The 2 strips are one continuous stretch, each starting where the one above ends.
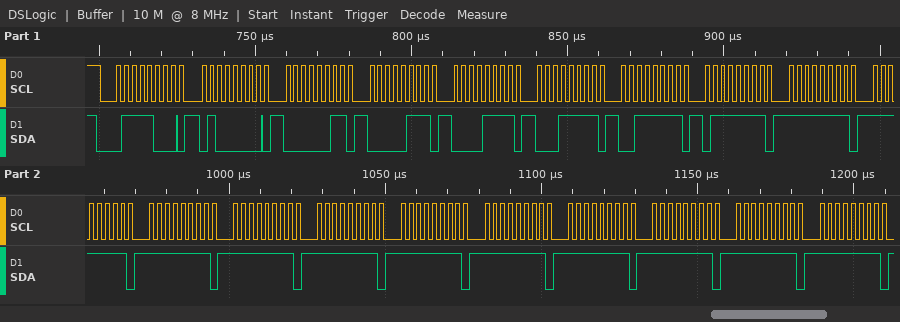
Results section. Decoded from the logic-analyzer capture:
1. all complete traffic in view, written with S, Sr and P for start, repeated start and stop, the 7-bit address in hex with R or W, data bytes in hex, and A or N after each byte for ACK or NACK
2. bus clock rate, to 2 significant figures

S 3CW A 40 A 03 A 07 A 0F A 1F A 3F A 7F A FF A FF A FF A FF A FF A FF A FF A FF A FF A FF A FF A
400 kHz
